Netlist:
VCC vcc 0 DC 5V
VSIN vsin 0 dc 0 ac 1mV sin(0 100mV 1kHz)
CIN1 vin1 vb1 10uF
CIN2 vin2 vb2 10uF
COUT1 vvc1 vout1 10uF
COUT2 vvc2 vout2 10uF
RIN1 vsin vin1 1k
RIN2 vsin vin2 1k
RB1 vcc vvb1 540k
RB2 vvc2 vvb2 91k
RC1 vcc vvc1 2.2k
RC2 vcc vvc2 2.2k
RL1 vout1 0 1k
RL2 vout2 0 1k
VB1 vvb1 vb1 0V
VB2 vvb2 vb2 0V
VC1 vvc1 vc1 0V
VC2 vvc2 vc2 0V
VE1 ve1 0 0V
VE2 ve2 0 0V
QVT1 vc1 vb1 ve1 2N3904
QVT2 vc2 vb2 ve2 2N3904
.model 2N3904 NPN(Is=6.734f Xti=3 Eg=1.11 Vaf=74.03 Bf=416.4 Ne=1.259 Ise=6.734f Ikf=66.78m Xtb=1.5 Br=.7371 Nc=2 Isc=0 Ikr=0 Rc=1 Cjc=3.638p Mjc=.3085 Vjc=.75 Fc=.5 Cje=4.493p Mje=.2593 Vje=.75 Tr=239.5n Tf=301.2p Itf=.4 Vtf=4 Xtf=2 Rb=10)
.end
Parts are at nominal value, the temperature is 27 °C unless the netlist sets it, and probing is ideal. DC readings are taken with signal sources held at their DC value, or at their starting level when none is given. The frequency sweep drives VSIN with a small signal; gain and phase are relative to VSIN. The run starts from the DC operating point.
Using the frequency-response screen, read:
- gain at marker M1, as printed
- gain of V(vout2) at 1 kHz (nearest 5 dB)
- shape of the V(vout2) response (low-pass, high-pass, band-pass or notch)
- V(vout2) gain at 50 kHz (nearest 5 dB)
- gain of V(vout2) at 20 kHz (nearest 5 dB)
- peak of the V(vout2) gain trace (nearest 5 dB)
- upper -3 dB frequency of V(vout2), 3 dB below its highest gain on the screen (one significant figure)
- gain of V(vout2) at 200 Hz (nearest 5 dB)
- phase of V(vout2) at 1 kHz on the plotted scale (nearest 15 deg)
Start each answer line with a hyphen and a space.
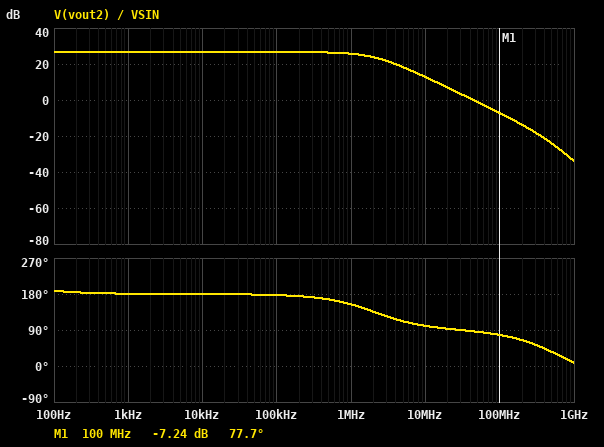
- -7.24 dB
- 25 dB
- low-pass
- 25 dB
- 25 dB
- 25 dB
- 2 MHz
- 25 dB
- 180 deg
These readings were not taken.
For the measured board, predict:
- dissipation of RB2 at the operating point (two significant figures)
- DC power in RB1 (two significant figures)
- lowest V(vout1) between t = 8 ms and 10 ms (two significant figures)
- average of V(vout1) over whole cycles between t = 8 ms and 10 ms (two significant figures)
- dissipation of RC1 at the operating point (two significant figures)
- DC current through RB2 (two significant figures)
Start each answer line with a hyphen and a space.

- 10 µW
- 35 µW
- -2.0 V
- -310 mV
- 2.7 mW
- 11 µA
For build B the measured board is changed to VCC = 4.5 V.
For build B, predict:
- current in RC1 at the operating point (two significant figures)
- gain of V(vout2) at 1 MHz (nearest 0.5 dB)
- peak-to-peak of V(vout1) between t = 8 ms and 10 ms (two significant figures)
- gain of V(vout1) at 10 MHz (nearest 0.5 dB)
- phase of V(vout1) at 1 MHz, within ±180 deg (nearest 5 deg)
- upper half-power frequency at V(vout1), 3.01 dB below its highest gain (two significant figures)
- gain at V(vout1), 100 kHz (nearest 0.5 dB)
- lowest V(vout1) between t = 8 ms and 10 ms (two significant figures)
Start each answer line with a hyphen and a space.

- 960 µA
- 25.0 dB
- 2.7 V
- 13.0 dB
- 155 deg
- 2.3 MHz
- 26.0 dB
- -1.9 V
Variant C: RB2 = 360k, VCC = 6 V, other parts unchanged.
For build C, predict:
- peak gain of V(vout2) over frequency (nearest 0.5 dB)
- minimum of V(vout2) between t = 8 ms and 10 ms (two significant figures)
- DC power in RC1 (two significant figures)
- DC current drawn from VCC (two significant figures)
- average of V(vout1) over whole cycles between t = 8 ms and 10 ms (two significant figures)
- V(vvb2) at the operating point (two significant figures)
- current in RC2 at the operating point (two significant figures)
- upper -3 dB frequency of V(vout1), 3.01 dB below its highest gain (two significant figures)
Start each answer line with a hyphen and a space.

- 26.5 dB
- -2.8 V
- 4.3 mW
- 2.5 mA
- -320 mV
- 670 mV
- 1.1 mA
- 1.9 MHz
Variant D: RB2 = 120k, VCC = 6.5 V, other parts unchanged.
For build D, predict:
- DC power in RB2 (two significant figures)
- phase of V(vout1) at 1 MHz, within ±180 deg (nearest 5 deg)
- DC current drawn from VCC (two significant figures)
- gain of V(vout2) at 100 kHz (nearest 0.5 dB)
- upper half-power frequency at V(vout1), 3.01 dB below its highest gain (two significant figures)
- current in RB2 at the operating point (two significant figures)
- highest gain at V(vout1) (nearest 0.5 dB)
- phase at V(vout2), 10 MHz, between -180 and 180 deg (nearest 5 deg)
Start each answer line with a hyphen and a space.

- 21 µW
- 150 deg
- 3.5 mA
- 28.5 dB
- 1.8 MHz
- 13 µA
- 29.5 dB
- 100 deg
